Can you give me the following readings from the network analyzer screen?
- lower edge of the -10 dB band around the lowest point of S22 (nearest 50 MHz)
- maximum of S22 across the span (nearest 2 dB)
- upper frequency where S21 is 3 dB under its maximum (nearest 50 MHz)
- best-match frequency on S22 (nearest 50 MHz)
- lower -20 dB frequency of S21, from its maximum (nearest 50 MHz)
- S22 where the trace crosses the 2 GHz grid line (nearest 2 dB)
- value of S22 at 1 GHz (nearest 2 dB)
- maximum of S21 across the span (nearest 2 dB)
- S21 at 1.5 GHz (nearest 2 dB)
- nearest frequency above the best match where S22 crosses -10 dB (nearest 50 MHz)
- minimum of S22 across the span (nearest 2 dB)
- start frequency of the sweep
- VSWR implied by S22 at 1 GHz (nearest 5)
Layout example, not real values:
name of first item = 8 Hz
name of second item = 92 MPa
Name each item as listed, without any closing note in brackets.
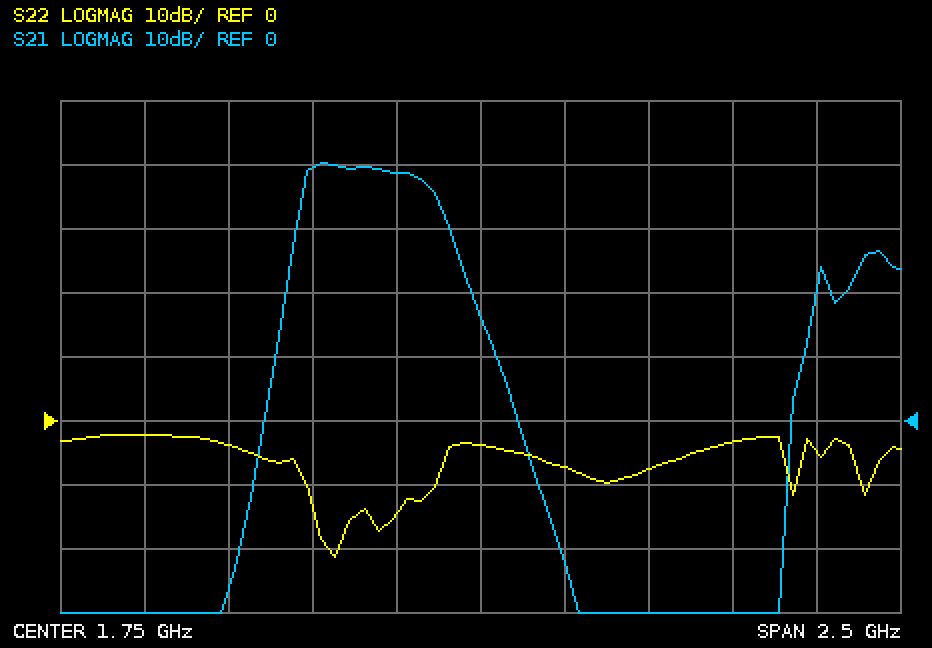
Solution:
lower edge of the -10 dB band around the lowest point of S22 = 1.25 GHz
maximum of S22 across the span = -2 dB
upper frequency where S21 is 3 dB under its maximum = 1.60 GHz
best-match frequency on S22 = 1.30 GHz
lower -20 dB frequency of S21, from its maximum = 1.15 GHz
S22 where the trace crosses the 2 GHz grid line = -8 dB
value of S22 at 1 GHz = -4 dB
maximum of S21 across the span = 40 dB
S21 at 1.5 GHz = 38 dB
nearest frequency above the best match where S22 crosses -10 dB = 1.60 GHz
minimum of S22 across the span = -22 dB
start frequency of the sweep = 500 MHz
VSWR implied by S22 at 1 GHz = 5
